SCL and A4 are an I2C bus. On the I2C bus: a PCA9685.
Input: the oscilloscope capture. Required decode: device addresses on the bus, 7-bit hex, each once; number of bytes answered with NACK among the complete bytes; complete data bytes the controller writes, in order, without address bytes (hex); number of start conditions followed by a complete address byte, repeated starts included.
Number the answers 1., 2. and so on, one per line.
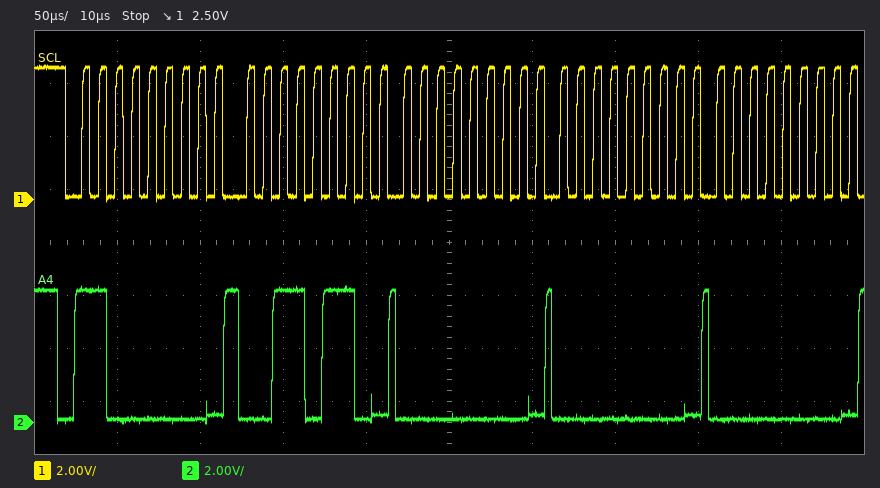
1. 0x60
2. 0
3. 36 00 00 00
4. 1
